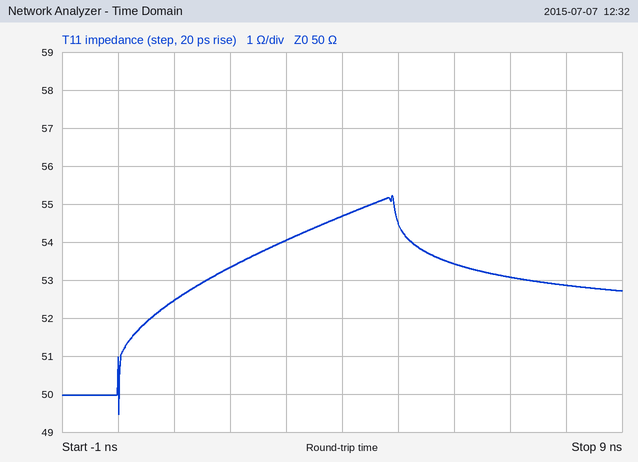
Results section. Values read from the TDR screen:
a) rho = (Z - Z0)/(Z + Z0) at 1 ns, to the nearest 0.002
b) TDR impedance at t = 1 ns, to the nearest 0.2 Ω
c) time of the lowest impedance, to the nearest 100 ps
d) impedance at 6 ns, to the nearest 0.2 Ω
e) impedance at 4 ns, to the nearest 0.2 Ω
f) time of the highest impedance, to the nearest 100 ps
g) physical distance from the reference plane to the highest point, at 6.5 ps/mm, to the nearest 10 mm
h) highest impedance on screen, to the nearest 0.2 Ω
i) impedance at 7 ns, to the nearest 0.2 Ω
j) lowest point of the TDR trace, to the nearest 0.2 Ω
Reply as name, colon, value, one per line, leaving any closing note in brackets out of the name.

rho = (Z - Z0)/(Z + Z0) at 1 ns, to the nearest 0.002: +0.024
TDR impedance at t = 1 ns, to the nearest 0.2 Ω: 52.4 Ω
time of the lowest impedance, to the nearest 100 ps: 0.0 ns
impedance at 6 ns, to the nearest 0.2 Ω: 53.4 Ω
impedance at 4 ns, to the nearest 0.2 Ω: 54.6 Ω
time of the highest impedance, to the nearest 100 ps: 4.9 ns
physical distance from the reference plane to the highest point, at 6.5 ps/mm, to the nearest 10 mm: 380 mm
highest impedance on screen, to the nearest 0.2 Ω: 55.2 Ω
impedance at 7 ns, to the nearest 0.2 Ω: 53.0 Ω
lowest point of the TDR trace, to the nearest 0.2 Ω: 49.4 Ω
